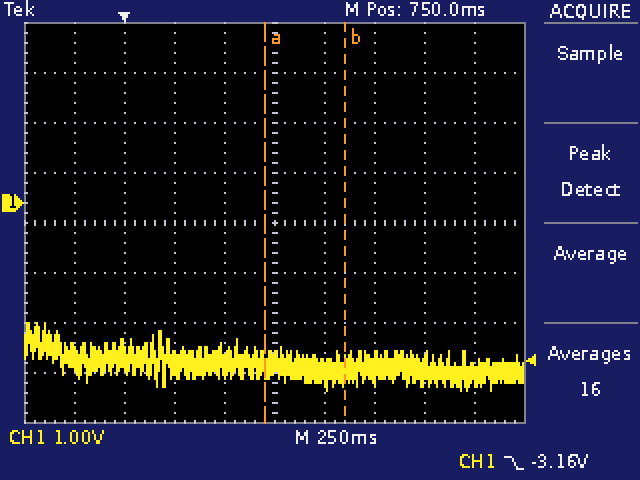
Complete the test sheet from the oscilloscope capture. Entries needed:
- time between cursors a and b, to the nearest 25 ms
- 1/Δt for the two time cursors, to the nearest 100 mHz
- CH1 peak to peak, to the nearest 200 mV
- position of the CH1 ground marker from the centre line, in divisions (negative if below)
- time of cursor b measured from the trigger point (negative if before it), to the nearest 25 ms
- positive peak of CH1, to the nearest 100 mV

400 ms
2.5 Hz
1.4 V
+0.4 div
+1.100 s
-2.4 V
